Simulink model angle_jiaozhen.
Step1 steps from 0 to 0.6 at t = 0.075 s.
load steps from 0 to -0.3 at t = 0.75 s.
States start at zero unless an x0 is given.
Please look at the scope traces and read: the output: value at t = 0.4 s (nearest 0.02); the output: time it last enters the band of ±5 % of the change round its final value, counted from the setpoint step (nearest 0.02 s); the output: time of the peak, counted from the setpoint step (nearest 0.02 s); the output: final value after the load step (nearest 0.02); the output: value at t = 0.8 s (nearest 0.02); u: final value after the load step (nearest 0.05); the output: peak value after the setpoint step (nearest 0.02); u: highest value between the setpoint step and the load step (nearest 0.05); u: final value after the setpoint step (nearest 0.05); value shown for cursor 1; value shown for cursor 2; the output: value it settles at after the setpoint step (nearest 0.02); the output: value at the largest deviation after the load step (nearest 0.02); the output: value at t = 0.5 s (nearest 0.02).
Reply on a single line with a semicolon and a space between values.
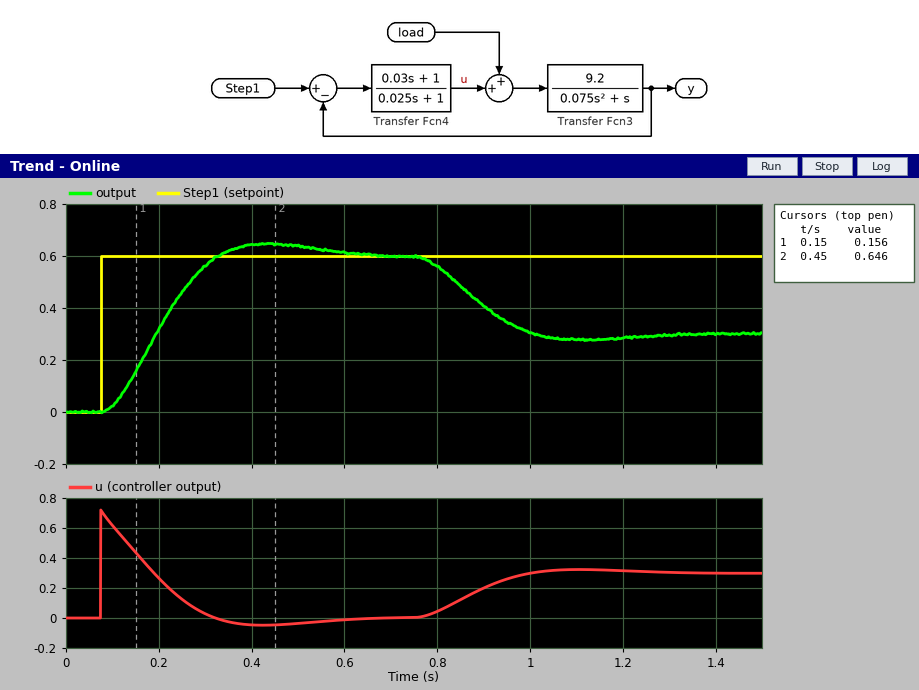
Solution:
0.64; 0.46 s; 0.36 s; 0.30; 0.56; 0.30; 0.64; 0.70; 0.00; 0.156; 0.646; 0.60; 0.28; 0.64
